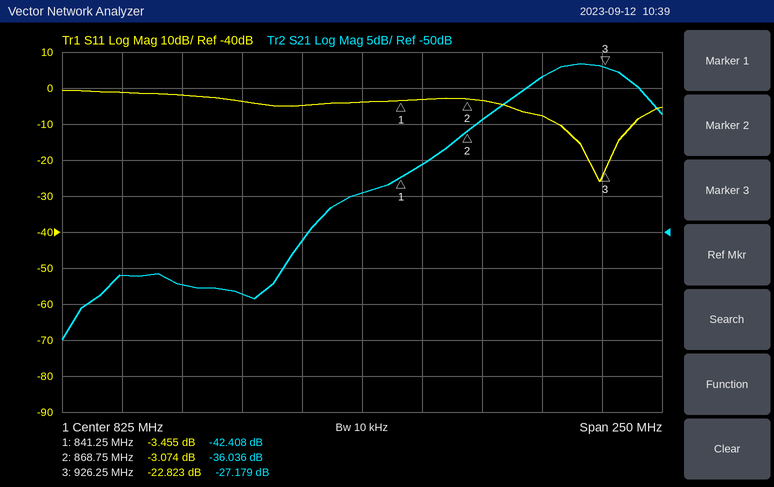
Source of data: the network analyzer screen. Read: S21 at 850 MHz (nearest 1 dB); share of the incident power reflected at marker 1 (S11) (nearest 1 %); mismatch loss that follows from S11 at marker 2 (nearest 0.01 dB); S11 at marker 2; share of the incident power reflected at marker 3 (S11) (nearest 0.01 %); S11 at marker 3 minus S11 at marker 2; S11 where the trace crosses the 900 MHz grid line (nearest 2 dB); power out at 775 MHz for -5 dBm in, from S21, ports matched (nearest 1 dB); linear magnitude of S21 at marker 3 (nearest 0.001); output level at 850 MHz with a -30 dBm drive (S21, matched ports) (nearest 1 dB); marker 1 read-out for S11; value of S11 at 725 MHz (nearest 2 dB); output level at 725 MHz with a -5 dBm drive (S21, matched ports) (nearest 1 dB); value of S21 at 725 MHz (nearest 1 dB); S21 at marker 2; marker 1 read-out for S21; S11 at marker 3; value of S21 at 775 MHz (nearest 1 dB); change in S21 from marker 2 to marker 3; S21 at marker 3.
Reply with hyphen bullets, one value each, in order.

- -41 dB
- 45 %
- 2.95 dB
- -3.074 dB
- 0.52 %
- -19.749 dB
- -8 dB
- -64 dBm
- 0.044
- -71 dBm
- -3.455 dB
- -2 dB
- -61 dBm
- -56 dB
- -36.036 dB
- -42.408 dB
- -22.823 dB
- -59 dB
- 8.857 dB
- -27.179 dB
